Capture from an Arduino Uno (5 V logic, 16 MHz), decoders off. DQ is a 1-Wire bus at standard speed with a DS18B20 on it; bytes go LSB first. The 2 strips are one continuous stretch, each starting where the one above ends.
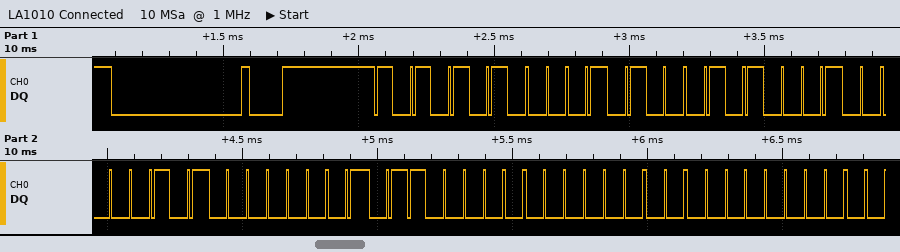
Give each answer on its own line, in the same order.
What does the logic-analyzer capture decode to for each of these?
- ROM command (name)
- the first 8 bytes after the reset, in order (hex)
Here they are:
Match ROM
55 28 8A A0 80 06 00 00
